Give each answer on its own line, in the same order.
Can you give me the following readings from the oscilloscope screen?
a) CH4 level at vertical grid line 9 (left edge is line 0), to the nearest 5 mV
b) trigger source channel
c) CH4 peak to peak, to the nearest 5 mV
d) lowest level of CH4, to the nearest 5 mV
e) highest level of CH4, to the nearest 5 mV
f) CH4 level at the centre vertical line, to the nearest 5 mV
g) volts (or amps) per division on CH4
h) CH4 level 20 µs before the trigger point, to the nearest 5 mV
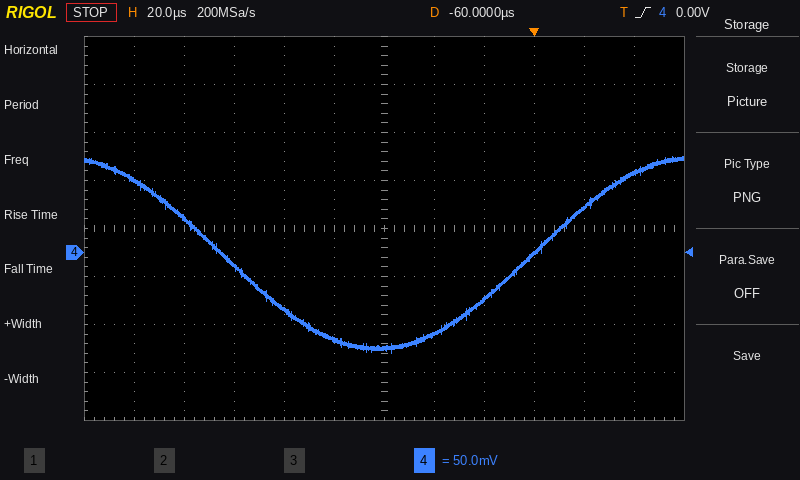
0 mV
CH4
205 mV
-105 mV
100 mV
-100 mV
50 mV
-50 mV
